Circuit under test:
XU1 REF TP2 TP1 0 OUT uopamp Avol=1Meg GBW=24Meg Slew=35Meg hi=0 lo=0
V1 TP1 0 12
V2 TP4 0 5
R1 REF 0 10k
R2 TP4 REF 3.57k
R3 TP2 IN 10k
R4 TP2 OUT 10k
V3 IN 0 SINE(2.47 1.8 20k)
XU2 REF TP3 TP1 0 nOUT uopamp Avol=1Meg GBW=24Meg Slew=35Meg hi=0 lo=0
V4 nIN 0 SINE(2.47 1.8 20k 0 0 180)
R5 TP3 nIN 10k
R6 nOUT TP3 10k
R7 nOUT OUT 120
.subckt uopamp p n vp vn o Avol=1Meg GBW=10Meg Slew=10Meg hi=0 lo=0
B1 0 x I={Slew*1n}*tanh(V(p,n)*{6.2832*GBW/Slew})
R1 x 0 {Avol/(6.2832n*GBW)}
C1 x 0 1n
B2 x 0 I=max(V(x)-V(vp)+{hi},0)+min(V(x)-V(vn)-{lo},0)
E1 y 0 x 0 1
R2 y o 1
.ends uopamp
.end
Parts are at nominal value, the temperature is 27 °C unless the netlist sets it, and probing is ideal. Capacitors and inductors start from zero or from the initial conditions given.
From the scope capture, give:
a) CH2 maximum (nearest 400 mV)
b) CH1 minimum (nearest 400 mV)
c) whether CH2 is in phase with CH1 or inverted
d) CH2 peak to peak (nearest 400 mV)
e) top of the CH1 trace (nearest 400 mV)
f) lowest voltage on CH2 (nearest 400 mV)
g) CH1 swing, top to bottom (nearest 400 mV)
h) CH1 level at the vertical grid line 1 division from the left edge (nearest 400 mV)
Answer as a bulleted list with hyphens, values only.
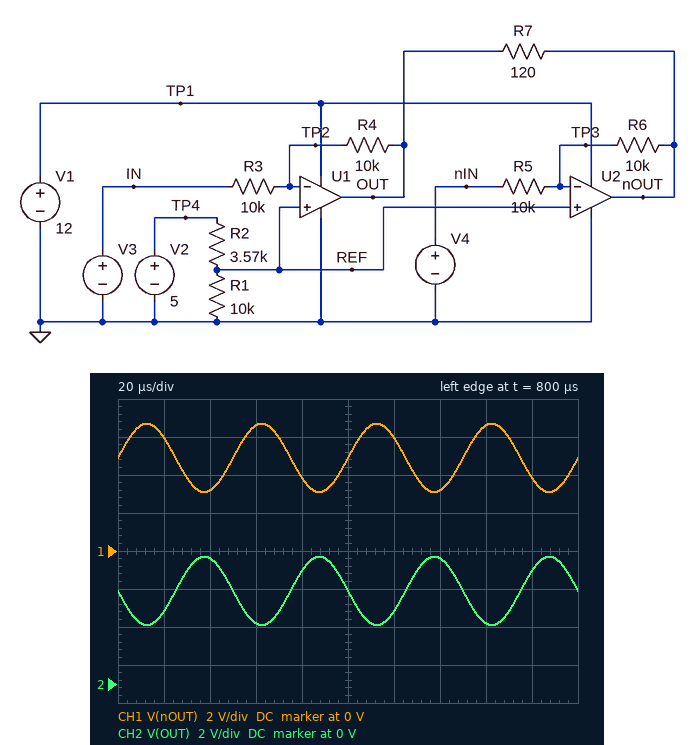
- 6.8 V
- 3.2 V
- inverted
- 3.6 V
- 6.8 V
- 3.2 V
- 3.6 V
- 6.0 V
